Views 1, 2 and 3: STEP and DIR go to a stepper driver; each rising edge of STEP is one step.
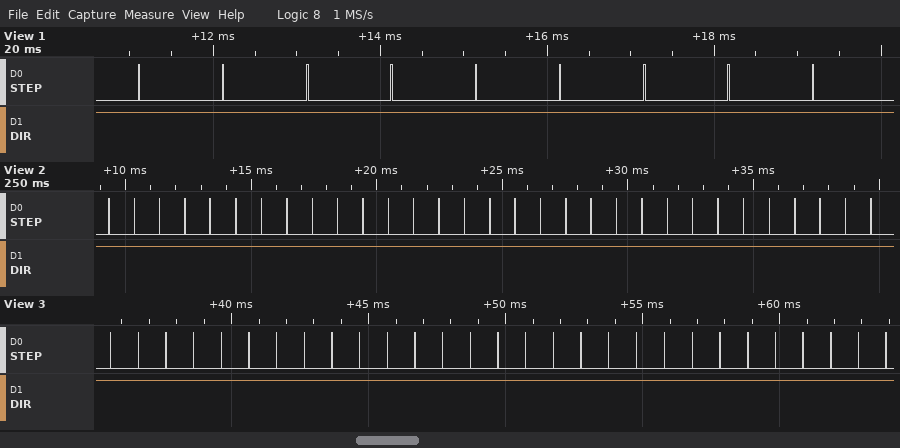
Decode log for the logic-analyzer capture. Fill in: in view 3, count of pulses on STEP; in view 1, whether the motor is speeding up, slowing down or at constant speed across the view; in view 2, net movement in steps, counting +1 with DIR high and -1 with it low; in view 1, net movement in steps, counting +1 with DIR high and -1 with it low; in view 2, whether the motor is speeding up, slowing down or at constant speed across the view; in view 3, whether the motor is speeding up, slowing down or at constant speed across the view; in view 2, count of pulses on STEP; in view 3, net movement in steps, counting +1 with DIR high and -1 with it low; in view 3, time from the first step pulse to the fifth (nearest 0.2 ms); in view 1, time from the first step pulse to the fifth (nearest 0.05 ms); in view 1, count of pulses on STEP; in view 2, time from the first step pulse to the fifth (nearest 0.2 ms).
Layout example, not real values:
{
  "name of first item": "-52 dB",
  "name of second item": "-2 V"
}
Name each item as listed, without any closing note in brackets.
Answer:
{
  "in view 3, count of pulses on STEP": "29",
  "in view 1, whether the motor is speeding up, slowing down or at constant speed across the view": "constant speed",
  "in view 2, net movement in steps, counting +1 with DIR high and -1 with it low": "+31",
  "in view 1, net movement in steps, counting +1 with DIR high and -1 with it low": "+9",
  "in view 2, whether the motor is speeding up, slowing down or at constant speed across the view": "constant speed",
  "in view 3, whether the motor is speeding up, slowing down or at constant speed across the view": "constant speed",
  "in view 2, count of pulses on STEP": "31",
  "in view 3, net movement in steps, counting +1 with DIR high and -1 with it low": "+29",
  "in view 3, time from the first step pulse to the fifth": "4.0 ms",
  "in view 1, time from the first step pulse to the fifth": "4.05 ms",
  "in view 1, count of pulses on STEP": "9",
  "in view 2, time from the first step pulse to the fifth": "4.0 ms"
}
